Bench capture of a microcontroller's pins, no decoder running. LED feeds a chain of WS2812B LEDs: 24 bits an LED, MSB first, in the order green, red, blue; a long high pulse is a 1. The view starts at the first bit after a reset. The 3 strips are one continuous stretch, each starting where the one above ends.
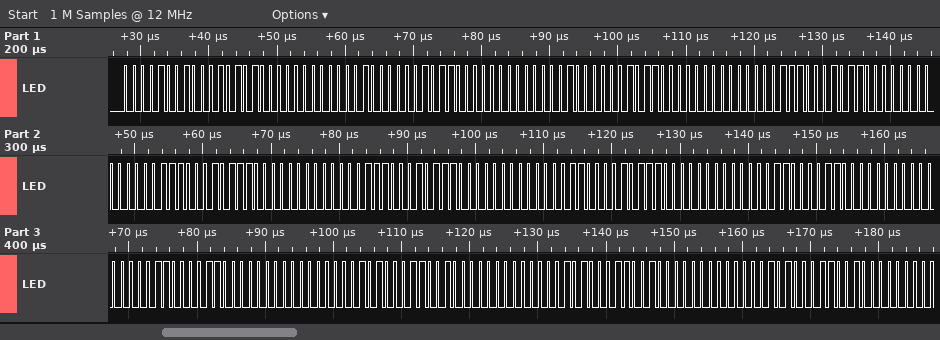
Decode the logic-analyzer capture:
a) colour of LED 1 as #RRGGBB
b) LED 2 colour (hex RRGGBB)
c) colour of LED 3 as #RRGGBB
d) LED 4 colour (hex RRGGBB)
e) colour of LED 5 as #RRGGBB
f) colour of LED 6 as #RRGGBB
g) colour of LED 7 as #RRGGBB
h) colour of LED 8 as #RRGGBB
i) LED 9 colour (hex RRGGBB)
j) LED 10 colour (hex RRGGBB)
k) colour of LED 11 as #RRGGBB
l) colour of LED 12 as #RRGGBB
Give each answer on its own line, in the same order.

#150900
#160800
#160800
#160700
#170700
#170700
#170600
#180600
#180600
#190500
#190500
#190500
